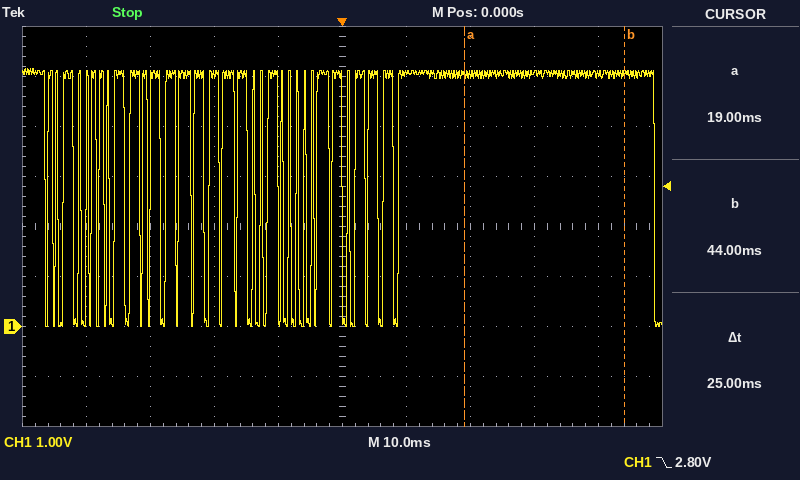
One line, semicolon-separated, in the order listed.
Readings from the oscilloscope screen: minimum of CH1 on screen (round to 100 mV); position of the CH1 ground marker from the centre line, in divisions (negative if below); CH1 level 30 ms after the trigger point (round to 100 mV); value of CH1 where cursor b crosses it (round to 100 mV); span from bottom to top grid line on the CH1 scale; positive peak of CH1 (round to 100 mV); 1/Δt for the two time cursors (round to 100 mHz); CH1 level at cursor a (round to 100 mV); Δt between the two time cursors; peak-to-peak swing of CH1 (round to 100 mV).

0.0 V; -2.0 div; 5.1 V; 5.0 V; 8 V; 5.2 V; 40.0 Hz; 5.0 V; 25 ms; 5.2 V
